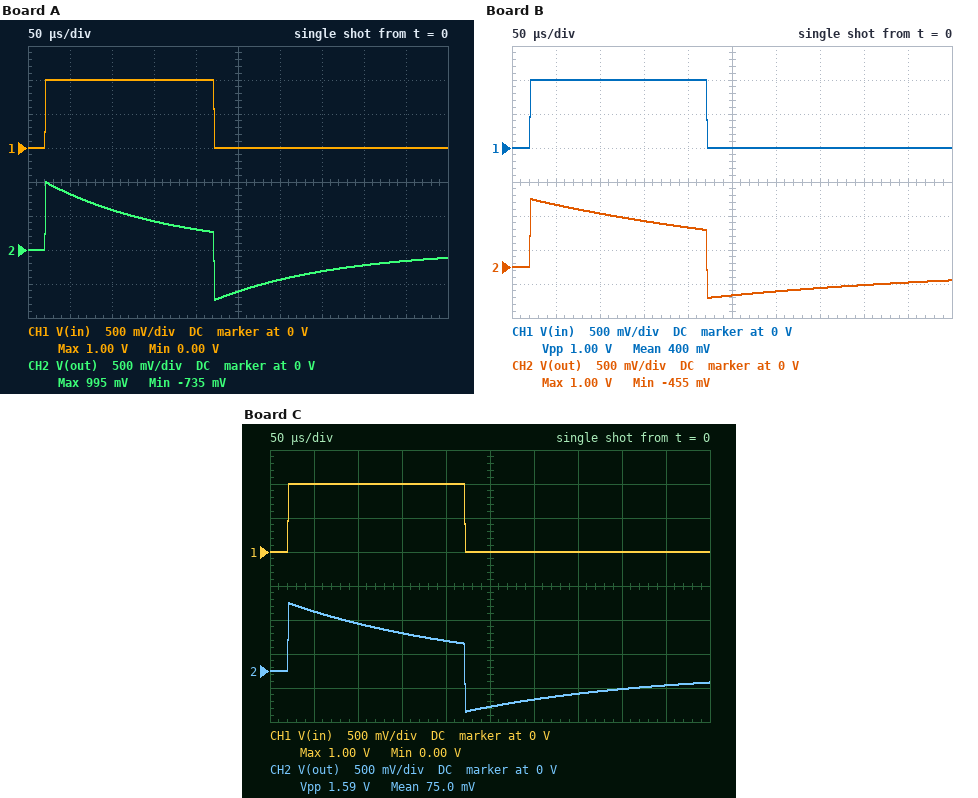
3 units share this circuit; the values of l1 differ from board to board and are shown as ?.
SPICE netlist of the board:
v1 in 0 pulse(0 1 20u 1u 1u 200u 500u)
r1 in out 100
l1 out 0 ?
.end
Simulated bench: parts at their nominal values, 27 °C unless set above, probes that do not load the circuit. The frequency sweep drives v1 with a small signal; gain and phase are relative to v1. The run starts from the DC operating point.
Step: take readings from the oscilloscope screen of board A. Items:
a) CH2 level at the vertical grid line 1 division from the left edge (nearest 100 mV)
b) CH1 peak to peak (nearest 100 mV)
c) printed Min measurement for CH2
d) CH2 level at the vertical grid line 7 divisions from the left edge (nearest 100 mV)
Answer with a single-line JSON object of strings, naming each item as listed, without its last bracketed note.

{"CH2 level at the vertical grid line 1 division from the left edge": "800 mV", "CH1 peak to peak": "1.0 V", "printed Min measurement for CH2": "-735 mV", "CH2 level at the vertical grid line 7 divisions from the left edge": "-300 mV"}
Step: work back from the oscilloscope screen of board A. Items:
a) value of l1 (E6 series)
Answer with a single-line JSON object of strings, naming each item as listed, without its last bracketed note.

{"value of l1": "15 mH"}
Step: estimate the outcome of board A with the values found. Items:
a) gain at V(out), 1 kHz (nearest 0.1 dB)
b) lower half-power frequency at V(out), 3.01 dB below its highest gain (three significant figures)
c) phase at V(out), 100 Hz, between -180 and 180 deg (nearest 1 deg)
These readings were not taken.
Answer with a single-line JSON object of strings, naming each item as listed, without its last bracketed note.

{"gain at V(out), 1 kHz": "-3.3 dB", "lower half-power frequency at V(out), 3.01 dB below its highest gain": "1.06 kHz", "phase at V(out), 100 Hz, between -180 and 180 deg": "85 deg"}
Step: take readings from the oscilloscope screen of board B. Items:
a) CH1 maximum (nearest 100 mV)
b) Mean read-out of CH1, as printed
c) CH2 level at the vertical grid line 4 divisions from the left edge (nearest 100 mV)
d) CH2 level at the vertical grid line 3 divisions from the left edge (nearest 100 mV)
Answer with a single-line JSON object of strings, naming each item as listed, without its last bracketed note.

{"CH1 maximum": "1.0 V", "Mean read-out of CH1, as printed": "400 mV", "CH2 level at the vertical grid line 4 divisions from the left edge": "600 mV", "CH2 level at the vertical grid line 3 divisions from the left edge": "700 mV"}
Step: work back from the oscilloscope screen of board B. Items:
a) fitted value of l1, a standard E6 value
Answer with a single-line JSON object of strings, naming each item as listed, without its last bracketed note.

{"fitted value of l1, a standard E6 value": "33 mH"}
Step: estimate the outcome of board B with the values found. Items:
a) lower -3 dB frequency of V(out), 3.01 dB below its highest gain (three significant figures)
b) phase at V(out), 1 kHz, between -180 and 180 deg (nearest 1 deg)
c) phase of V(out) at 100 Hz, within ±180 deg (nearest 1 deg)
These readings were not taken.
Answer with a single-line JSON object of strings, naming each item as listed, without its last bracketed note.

{"lower -3 dB frequency of V(out), 3.01 dB below its highest gain": "482 Hz", "phase at V(out), 1 kHz, between -180 and 180 deg": "26 deg", "phase of V(out) at 100 Hz, within ±180 deg": "78 deg"}
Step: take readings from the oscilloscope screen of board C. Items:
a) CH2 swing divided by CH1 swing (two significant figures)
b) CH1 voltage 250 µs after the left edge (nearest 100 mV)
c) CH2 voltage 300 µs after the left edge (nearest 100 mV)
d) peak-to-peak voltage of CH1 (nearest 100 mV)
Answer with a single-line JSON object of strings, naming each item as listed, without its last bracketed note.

{"CH2 swing divided by CH1 swing": "1.6", "CH1 voltage 250 µs after the left edge": "0 V", "CH2 voltage 300 µs after the left edge": "-400 mV", "peak-to-peak voltage of CH1": "1.0 V"}
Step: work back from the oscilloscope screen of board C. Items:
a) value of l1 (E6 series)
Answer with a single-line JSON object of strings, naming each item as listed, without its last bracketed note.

{"value of l1": "22 mH"}
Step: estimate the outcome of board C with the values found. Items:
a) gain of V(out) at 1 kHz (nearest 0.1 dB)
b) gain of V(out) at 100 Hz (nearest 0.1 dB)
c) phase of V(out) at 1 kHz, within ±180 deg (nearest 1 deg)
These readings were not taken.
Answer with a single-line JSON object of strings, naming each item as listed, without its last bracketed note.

{"gain of V(out) at 1 kHz": "-1.8 dB", "gain of V(out) at 100 Hz": "-17.3 dB", "phase of V(out) at 1 kHz, within ±180 deg": "36 deg"}
